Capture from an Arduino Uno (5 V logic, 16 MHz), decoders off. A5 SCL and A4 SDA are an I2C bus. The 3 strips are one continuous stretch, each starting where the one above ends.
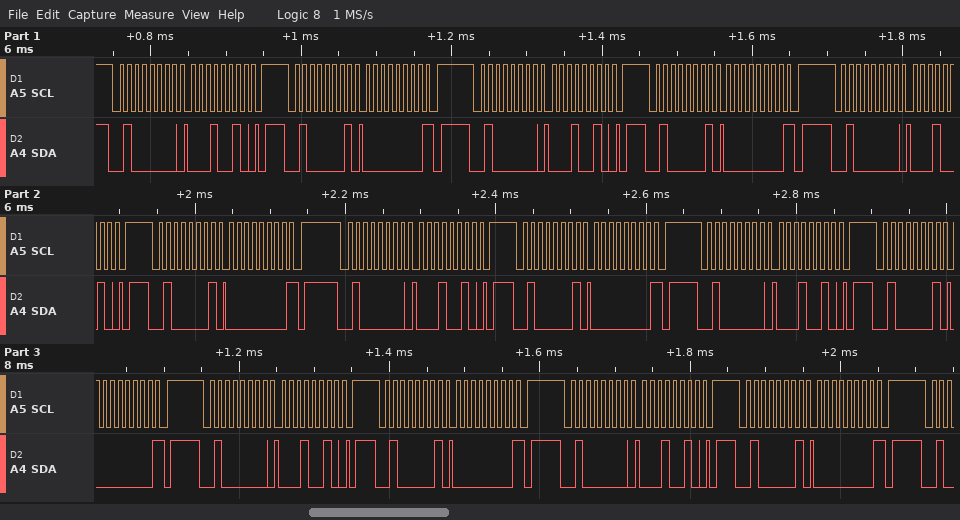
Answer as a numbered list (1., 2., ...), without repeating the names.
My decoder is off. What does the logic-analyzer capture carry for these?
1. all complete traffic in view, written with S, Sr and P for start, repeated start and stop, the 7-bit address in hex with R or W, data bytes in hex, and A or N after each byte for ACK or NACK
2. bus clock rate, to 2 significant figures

1. S 20W A 12 A P S 20R A 00 N P S 20W A 12 A P S 20R A 00 N P S 20W A 12 A P S 20R A 00 N P S 20W A 12 A P S 20R A 00 N P S 20W A 12 A P S 20R A 00 N P S 20W A 12 A P S 20R A 00 N P S 20W A 12 A P S 20R A 00 N P
2. 100 kHz
